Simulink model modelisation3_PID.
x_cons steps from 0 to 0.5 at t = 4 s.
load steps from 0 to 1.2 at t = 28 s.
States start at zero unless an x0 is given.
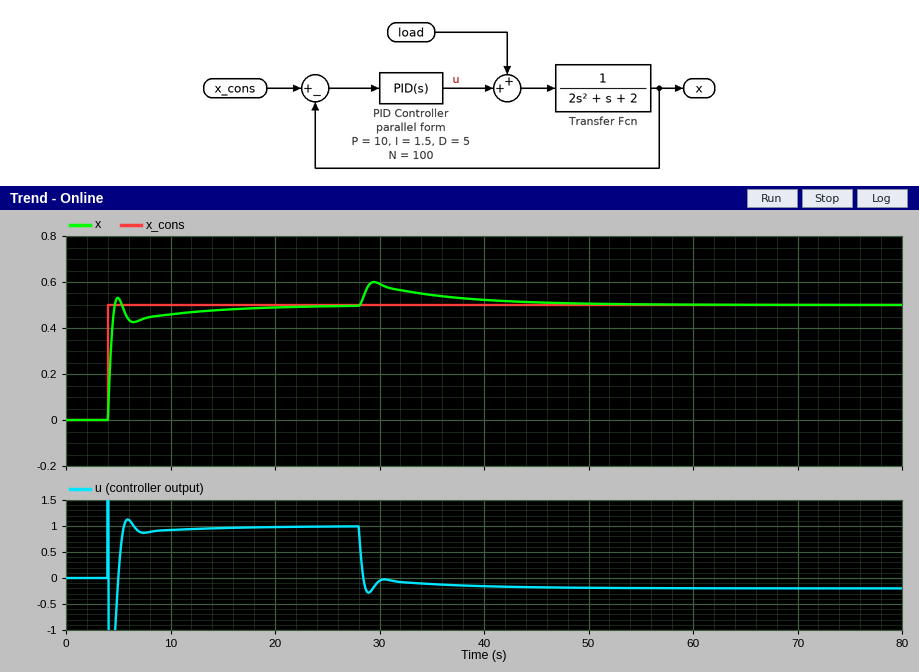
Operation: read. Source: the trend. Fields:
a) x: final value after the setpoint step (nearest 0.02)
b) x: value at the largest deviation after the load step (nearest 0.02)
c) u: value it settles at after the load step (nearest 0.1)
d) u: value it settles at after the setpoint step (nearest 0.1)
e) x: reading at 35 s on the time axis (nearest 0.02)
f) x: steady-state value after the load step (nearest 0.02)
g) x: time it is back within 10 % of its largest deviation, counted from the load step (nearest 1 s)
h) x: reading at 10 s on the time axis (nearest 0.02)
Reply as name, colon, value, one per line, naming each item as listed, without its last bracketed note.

x: final value after the setpoint step: 0.50
x: value at the largest deviation after the load step: 0.60
u: value it settles at after the load step: -0.2
u: value it settles at after the setpoint step: 1.0
x: reading at 35 s on the time axis: 0.54
x: steady-state value after the load step: 0.50
x: time it is back within 10 % of its largest deviation, counted from the load step: 18 s
x: reading at 10 s on the time axis: 0.46
